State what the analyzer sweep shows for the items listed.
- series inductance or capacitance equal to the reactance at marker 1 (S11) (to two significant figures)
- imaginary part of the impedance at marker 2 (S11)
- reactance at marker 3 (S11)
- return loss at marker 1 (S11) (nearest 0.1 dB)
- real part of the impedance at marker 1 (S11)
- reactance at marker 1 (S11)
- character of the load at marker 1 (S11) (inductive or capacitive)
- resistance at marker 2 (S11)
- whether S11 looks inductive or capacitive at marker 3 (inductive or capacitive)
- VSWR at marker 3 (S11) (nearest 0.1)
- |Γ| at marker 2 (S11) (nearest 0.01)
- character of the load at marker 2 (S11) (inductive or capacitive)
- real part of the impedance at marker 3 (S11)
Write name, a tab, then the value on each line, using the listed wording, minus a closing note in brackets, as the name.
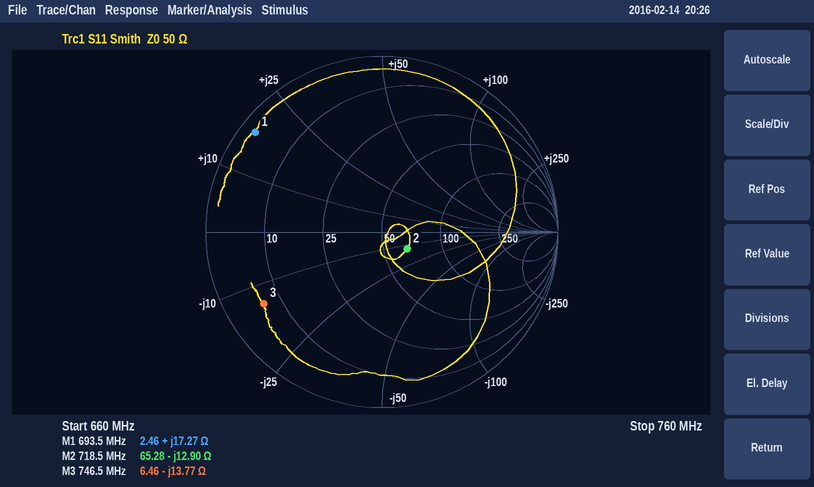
series inductance or capacitance equal to the reactance at marker 1 (S11)	4.0 nH
imaginary part of the impedance at marker 2	-12.90 Ω
reactance at marker 3	-13.77 Ω
return loss at marker 1 (S11)	0.8 dB
real part of the impedance at marker 1	2.46 Ω
reactance at marker 1	+17.27 Ω
character of the load at marker 1 (S11)	inductive
resistance at marker 2	65.28 Ω
whether S11 looks inductive or capacitive at marker 3	capacitive
VSWR at marker 3 (S11)	8.3
|Γ| at marker 2 (S11)	0.17
character of the load at marker 2 (S11)	capacitive
real part of the impedance at marker 3	6.46 Ω
